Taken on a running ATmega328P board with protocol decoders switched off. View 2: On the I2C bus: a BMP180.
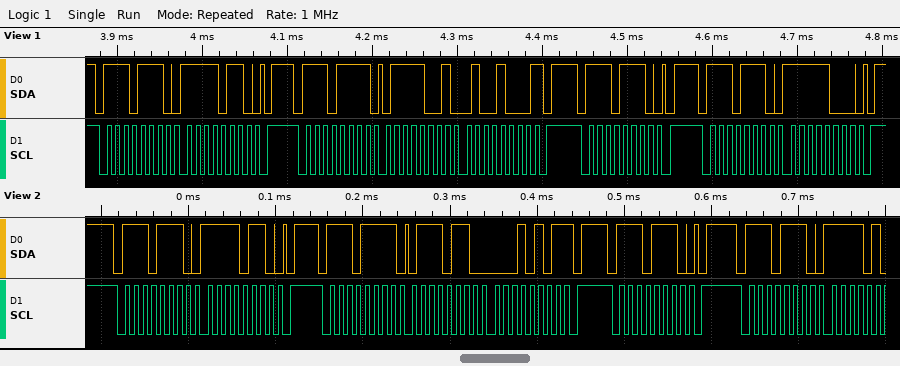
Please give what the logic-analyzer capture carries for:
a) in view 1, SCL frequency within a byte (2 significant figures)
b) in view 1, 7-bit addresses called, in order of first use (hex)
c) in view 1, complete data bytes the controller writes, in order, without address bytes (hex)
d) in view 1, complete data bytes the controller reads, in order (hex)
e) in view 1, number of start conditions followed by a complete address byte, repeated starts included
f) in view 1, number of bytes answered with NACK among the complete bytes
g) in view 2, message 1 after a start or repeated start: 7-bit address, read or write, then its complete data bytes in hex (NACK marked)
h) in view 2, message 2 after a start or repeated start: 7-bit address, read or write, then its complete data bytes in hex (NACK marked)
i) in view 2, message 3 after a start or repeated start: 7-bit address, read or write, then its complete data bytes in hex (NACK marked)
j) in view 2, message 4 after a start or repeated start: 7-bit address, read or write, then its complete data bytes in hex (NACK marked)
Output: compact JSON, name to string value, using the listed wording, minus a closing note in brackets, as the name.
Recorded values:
{"in view 1, SCL frequency within a byte": "100 kHz", "in view 1, 7-bit addresses called, in order of first use": "0x77", "in view 1, complete data bytes the controller writes, in order, without address bytes": "F6 F8", "in view 1, complete data bytes the controller reads, in order": "79 48", "in view 1, number of start conditions followed by a complete address byte, repeated starts included": "4", "in view 1, number of bytes answered with NACK among the complete bytes": "1", "in view 2, message 1 after a start or repeated start: 7-bit address, read or write, then its complete data bytes in hex": "0x77 write: F6", "in view 2, message 2 after a start or repeated start: 7-bit address, read or write, then its complete data bytes in hex": "0x77 read: 76 15 NACK", "in view 2, message 3 after a start or repeated start: 7-bit address, read or write, then its complete data bytes in hex": "0x77 write", "in view 2, message 4 after a start or repeated start: 7-bit address, read or write, then its complete data bytes in hex": "0x77 write"}
